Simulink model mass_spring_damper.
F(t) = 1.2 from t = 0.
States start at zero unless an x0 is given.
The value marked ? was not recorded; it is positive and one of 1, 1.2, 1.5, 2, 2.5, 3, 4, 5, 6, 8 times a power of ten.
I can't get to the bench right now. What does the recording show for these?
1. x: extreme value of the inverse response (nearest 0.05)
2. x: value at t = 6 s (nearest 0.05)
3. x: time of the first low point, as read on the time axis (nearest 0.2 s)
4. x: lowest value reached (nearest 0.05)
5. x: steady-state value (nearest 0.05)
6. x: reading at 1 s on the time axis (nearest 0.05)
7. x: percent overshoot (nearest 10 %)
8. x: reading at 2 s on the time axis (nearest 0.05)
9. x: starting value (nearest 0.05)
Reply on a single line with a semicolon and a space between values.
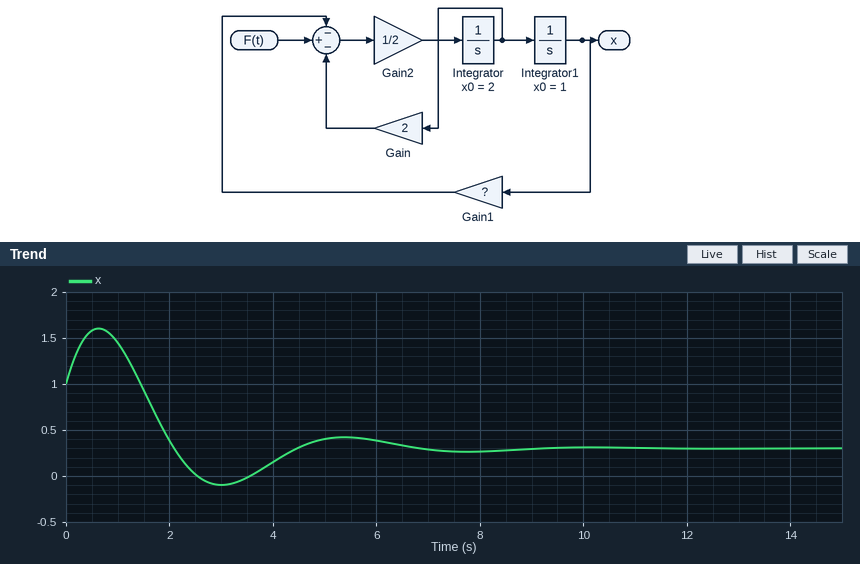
1.60; 0.40; 3.0 s; -0.10; 0.30; 1.45; 60 %; 0.40; 1.00
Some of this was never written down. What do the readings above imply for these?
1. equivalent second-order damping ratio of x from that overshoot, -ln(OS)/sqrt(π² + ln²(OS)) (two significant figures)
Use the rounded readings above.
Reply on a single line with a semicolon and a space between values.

0.16
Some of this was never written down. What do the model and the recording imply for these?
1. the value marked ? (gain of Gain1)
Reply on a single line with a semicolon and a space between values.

4
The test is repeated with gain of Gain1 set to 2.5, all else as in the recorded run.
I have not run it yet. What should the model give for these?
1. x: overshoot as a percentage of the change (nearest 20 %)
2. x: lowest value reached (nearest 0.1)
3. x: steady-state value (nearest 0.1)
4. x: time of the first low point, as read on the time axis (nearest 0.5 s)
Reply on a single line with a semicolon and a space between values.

60 %; 0.2; 0.5; 4.0 s
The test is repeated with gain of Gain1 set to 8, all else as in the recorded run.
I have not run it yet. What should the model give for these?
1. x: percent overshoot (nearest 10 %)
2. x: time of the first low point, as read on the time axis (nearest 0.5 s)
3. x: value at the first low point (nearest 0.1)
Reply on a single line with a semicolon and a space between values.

60 %; 2.0 s; -0.4
